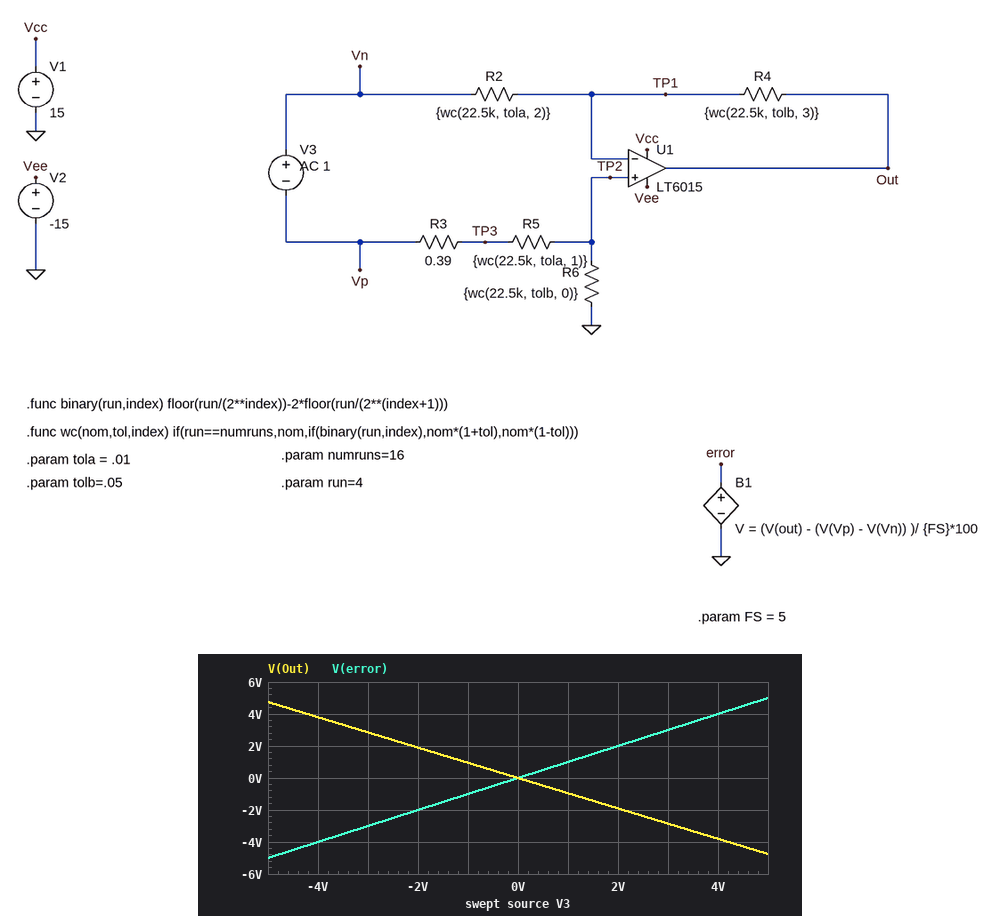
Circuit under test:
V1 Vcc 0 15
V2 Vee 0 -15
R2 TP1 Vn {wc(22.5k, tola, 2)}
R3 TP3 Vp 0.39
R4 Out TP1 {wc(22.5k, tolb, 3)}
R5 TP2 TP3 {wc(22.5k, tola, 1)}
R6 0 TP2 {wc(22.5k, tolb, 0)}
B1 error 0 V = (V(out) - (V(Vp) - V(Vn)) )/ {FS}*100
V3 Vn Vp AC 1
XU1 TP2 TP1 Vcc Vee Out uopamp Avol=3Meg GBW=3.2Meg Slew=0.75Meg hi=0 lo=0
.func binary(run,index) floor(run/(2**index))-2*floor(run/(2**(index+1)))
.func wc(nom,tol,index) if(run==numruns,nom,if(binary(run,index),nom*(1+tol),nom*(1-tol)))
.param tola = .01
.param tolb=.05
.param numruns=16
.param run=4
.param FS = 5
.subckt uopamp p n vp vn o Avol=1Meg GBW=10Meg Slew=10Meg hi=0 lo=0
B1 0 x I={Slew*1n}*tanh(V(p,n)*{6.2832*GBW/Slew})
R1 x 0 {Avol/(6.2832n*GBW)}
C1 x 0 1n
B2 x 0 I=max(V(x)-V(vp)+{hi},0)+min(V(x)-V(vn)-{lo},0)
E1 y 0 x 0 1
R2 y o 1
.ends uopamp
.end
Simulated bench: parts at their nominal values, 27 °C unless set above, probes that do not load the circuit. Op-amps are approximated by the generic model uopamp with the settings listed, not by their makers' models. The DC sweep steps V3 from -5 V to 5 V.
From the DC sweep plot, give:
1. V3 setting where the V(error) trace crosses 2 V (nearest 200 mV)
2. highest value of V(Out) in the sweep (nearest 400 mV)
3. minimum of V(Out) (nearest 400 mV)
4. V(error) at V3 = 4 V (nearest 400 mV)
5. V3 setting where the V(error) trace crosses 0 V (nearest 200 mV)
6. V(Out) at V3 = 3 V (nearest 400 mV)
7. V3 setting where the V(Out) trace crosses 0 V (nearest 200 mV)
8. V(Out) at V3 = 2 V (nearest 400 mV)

2.0 V
4.8 V
-4.8 V
4.0 V
0 V
-2.8 V
0 V
-2.0 V
